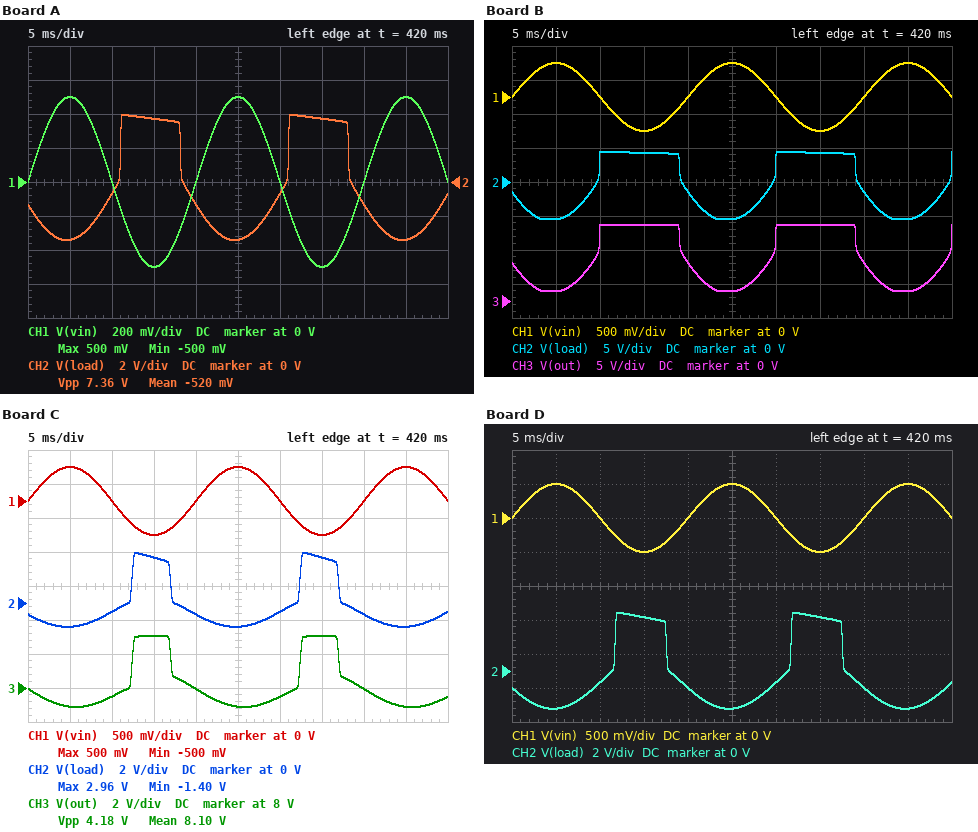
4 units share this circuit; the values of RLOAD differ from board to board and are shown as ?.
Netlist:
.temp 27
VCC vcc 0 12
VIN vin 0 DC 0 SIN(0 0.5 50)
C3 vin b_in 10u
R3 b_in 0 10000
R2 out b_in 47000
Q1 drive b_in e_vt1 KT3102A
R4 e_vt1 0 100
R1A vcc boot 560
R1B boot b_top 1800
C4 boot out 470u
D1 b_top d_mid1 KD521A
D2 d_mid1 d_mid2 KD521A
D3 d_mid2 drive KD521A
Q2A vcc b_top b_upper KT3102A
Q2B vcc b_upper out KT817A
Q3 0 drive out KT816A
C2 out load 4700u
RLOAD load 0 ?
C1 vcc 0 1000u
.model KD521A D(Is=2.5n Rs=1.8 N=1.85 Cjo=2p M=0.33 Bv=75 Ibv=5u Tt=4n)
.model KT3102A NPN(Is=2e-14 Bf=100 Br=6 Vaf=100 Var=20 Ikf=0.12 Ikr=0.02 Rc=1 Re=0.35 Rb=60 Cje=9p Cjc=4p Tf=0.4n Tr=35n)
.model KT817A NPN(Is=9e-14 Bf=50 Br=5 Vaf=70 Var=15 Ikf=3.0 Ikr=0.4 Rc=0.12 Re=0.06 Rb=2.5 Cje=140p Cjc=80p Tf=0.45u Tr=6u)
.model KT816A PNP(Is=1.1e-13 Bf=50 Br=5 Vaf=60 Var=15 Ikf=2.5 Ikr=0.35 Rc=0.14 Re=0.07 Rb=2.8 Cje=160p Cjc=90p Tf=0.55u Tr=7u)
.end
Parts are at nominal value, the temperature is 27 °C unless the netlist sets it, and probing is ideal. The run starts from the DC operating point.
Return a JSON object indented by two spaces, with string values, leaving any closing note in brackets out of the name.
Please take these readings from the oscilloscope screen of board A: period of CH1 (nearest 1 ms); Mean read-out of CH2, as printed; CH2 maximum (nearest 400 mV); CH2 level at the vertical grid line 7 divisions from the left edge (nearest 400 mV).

{
  "period of CH1": "20 ms",
  "Mean read-out of CH2, as printed": "-520 mV",
  "CH2 maximum": "4.0 V",
  "CH2 level at the vertical grid line 7 divisions from the left edge": "3.6 V"
}
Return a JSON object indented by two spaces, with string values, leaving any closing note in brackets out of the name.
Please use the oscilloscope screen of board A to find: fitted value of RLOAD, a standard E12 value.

{
  "fitted value of RLOAD, a standard E12 value": "12 Ω"
}
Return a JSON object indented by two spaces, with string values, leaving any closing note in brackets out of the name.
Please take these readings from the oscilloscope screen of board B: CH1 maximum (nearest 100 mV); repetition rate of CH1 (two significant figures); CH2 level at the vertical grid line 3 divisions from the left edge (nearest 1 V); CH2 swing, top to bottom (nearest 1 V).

{
  "CH1 maximum": "500 mV",
  "repetition rate of CH1": "50 Hz",
  "CH2 level at the vertical grid line 3 divisions from the left edge": "4 V",
  "CH2 swing, top to bottom": "10 V"
}
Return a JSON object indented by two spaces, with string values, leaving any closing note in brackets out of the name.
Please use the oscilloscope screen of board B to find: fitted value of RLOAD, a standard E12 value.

{
  "fitted value of RLOAD, a standard E12 value": "27 Ω"
}
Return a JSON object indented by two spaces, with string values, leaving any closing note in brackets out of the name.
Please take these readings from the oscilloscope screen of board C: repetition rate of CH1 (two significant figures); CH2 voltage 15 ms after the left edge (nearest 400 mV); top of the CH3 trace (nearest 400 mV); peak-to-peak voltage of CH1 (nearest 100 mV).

{
  "repetition rate of CH1": "50 Hz",
  "CH2 voltage 15 ms after the left edge": "2.8 V",
  "top of the CH3 trace": "11.2 V",
  "peak-to-peak voltage of CH1": "1.0 V"
}
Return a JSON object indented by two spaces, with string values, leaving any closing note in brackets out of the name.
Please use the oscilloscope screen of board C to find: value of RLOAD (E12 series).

{
  "value of RLOAD": "3.9 Ω"
}
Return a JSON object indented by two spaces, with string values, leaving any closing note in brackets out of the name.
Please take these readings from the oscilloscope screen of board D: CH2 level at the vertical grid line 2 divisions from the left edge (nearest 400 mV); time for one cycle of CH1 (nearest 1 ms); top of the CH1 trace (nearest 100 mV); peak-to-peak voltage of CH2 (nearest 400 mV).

{
  "CH2 level at the vertical grid line 2 divisions from the left edge": "-800 mV",
  "time for one cycle of CH1": "20 ms",
  "top of the CH1 trace": "500 mV",
  "peak-to-peak voltage of CH2": "5.6 V"
}
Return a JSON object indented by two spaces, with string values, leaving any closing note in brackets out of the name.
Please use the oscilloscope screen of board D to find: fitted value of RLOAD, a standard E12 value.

{
  "fitted value of RLOAD, a standard E12 value": "6.8 Ω"
}
